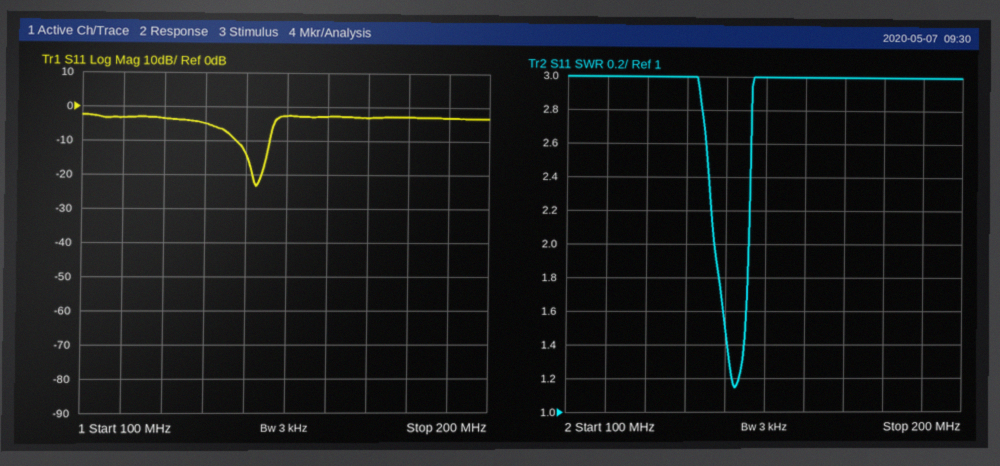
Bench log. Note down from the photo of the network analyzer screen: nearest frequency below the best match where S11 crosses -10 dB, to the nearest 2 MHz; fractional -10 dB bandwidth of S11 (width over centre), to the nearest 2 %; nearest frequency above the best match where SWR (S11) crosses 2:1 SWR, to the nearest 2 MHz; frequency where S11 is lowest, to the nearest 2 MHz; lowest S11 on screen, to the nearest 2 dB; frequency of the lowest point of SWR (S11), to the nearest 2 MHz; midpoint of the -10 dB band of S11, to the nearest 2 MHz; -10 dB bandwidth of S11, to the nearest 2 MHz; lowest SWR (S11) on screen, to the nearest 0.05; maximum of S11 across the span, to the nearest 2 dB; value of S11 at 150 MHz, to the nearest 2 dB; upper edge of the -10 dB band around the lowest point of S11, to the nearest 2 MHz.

138 MHz
6 %
146 MHz
142 MHz
-24 dB
142 MHz
142 MHz
8 MHz
1.15
-2 dB
-2 dB
146 MHz
